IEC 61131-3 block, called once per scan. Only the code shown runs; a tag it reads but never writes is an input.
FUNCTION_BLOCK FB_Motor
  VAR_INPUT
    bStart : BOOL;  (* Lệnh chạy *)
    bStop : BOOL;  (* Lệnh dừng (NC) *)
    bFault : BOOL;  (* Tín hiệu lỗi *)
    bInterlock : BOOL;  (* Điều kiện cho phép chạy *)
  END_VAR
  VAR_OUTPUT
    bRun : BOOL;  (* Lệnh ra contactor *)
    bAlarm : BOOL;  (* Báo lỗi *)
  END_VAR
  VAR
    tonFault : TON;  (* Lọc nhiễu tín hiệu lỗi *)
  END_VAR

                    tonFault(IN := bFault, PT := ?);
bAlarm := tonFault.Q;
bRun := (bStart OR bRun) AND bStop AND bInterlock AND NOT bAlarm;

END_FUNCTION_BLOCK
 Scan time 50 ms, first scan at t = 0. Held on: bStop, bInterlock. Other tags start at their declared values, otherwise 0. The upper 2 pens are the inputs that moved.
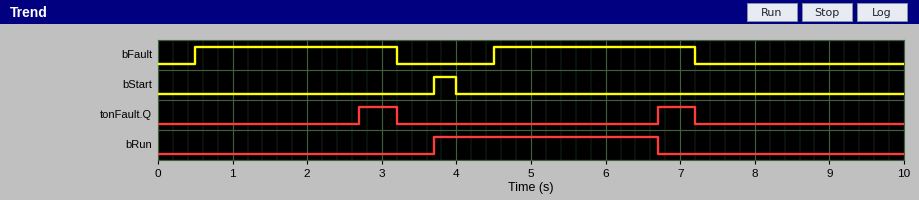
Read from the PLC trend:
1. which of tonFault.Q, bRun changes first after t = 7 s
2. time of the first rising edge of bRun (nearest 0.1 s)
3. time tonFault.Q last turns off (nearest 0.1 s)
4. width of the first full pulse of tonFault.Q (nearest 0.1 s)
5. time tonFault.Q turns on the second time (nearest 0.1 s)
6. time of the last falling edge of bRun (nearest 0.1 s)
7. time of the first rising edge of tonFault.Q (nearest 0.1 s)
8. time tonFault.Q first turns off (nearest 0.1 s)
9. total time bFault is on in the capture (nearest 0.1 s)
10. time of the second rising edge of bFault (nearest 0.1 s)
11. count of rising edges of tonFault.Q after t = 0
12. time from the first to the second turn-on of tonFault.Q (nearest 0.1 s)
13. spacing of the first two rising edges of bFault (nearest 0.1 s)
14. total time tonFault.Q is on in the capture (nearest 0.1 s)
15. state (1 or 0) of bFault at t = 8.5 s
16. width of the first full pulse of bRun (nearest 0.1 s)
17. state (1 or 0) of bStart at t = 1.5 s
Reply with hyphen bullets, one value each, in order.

- tonFault.Q
- 3.7 s
- 7.2 s
- 0.5 s
- 6.7 s
- 6.7 s
- 2.7 s
- 3.2 s
- 5.4 s
- 4.5 s
- 2
- 4.0 s
- 4.0 s
- 1.0 s
- 0
- 3.0 s
- 0
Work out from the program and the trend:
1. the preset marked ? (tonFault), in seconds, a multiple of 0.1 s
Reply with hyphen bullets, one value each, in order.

- 2.2 s
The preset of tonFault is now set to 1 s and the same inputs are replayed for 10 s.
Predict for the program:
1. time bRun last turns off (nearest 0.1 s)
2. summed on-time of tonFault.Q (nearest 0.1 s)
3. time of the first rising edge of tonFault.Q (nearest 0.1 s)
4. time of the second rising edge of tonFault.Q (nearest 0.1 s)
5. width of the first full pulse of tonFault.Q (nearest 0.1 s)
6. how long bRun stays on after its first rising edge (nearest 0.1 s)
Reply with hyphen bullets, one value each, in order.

- 5.5 s
- 3.4 s
- 1.5 s
- 5.5 s
- 1.7 s
- 1.8 s
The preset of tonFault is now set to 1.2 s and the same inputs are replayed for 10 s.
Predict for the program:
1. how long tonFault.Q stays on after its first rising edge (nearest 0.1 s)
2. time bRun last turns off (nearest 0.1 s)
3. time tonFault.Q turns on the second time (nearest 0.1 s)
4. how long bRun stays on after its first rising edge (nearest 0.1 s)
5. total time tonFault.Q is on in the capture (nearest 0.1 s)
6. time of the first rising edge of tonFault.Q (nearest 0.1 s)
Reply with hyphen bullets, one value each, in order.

- 1.5 s
- 5.7 s
- 5.7 s
- 2.0 s
- 3.0 s
- 1.7 s
